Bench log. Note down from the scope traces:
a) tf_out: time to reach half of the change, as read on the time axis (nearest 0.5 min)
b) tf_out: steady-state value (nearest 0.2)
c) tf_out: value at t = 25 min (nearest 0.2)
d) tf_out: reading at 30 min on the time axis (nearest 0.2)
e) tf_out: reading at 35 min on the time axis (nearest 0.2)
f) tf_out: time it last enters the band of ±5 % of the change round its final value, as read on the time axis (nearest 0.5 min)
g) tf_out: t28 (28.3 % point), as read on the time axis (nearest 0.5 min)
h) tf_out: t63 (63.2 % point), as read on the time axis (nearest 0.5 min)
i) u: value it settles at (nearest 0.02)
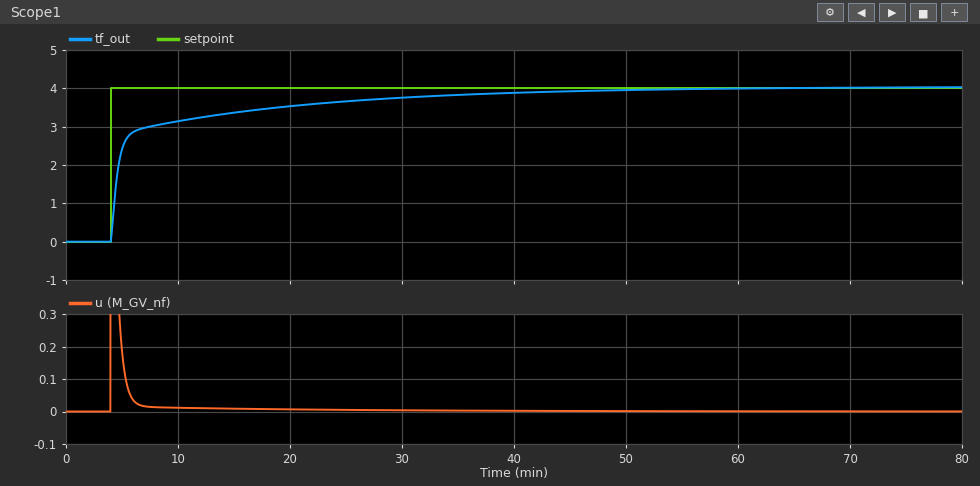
4.5 min
4.0
3.6
3.8
3.8
34.5 min
4.5 min
5.0 min
0.00
